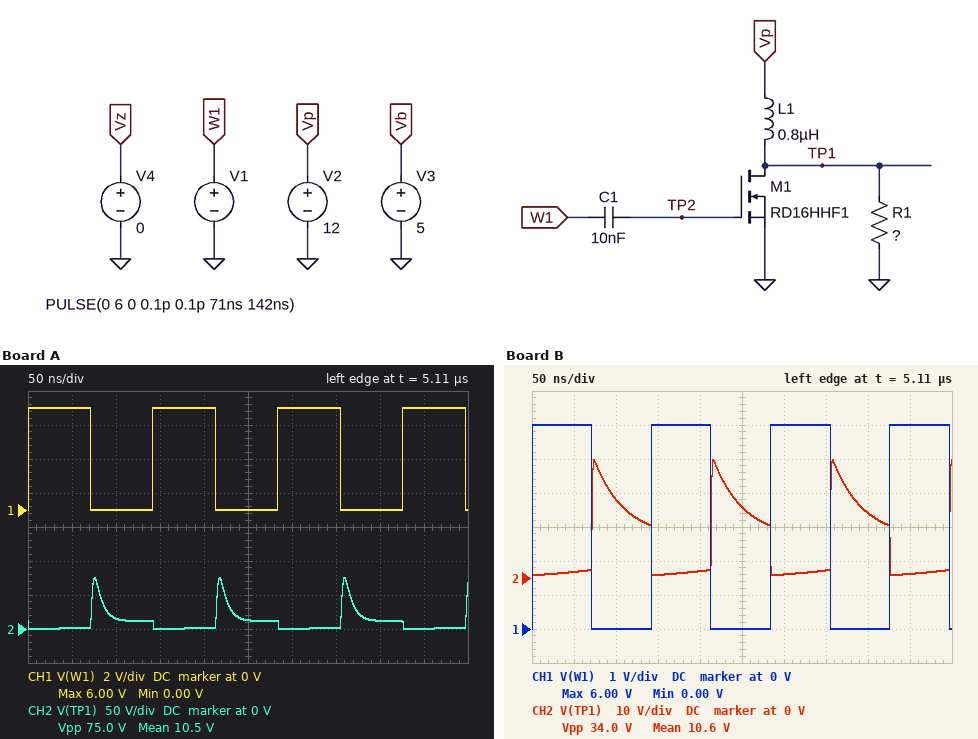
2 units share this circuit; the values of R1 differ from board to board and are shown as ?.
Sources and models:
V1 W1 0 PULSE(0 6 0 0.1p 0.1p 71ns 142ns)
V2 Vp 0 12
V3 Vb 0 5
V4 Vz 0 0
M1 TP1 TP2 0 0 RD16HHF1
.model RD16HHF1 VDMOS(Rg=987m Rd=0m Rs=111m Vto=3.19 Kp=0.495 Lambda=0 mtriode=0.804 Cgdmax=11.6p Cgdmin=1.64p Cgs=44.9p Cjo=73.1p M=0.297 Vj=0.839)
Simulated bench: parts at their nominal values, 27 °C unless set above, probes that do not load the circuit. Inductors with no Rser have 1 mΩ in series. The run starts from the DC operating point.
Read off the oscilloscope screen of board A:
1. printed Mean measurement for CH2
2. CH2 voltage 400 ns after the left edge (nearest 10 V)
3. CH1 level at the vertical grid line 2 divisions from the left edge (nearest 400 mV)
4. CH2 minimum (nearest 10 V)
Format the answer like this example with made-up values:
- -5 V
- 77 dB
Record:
- 10.5 V
- 10 V
- 0 V
- 0 V
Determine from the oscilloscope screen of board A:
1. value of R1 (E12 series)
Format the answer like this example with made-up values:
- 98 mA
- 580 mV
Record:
- 82 Ω
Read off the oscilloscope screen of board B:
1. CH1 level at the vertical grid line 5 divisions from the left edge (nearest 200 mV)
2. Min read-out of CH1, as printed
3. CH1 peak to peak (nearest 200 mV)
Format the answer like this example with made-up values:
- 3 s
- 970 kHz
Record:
- 0 V
- 0.00 V
- 6.0 V
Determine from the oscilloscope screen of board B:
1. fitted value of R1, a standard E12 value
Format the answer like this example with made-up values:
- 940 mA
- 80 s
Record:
- 22 Ω
